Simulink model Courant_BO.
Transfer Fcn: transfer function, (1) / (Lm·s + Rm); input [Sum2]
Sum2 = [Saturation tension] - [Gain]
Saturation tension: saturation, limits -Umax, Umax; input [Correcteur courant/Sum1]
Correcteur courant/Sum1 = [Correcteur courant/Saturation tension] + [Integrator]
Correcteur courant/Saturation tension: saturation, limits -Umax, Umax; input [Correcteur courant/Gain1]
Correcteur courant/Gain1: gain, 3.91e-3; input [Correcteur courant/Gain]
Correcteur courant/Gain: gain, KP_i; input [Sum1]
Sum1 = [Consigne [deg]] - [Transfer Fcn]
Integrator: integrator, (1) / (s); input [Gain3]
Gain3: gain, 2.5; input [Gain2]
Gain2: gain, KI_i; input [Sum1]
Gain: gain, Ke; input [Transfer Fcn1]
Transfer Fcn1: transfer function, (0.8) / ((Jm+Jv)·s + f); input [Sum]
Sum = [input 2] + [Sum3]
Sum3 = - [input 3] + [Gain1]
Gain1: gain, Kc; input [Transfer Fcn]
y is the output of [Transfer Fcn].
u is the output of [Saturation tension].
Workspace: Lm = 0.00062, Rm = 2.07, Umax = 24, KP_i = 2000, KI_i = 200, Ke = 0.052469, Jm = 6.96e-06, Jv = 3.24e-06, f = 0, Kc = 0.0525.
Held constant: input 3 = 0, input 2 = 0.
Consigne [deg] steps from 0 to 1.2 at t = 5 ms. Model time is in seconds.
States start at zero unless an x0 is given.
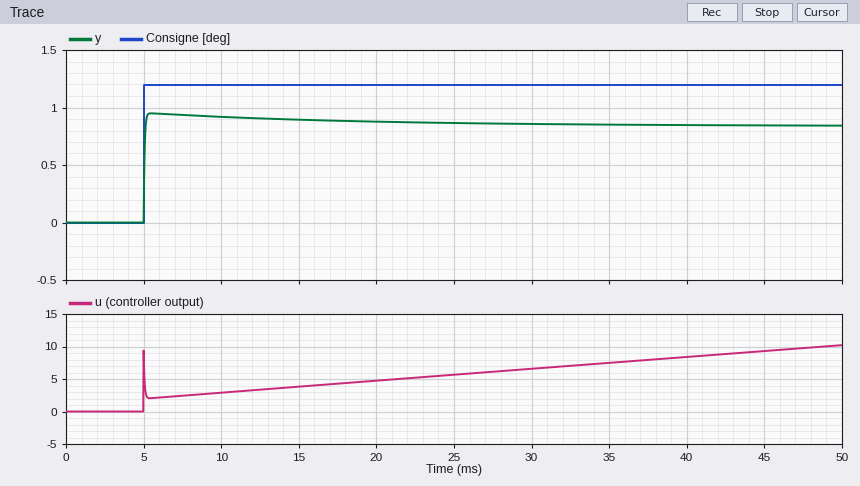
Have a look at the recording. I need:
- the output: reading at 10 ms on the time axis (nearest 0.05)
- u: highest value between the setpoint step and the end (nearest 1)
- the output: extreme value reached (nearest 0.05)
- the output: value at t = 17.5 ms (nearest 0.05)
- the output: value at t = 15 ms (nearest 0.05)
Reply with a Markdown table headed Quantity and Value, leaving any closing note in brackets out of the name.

| Quantity | Value |
|---|---|
| the output: reading at 10 ms on the time axis | 0.90 |
| u: highest value between the setpoint step and the end | 10 |
| the output: extreme value reached | 0.95 |
| the output: value at t = 17.5 ms | 0.90 |
| the output: value at t = 15 ms | 0.90 |
